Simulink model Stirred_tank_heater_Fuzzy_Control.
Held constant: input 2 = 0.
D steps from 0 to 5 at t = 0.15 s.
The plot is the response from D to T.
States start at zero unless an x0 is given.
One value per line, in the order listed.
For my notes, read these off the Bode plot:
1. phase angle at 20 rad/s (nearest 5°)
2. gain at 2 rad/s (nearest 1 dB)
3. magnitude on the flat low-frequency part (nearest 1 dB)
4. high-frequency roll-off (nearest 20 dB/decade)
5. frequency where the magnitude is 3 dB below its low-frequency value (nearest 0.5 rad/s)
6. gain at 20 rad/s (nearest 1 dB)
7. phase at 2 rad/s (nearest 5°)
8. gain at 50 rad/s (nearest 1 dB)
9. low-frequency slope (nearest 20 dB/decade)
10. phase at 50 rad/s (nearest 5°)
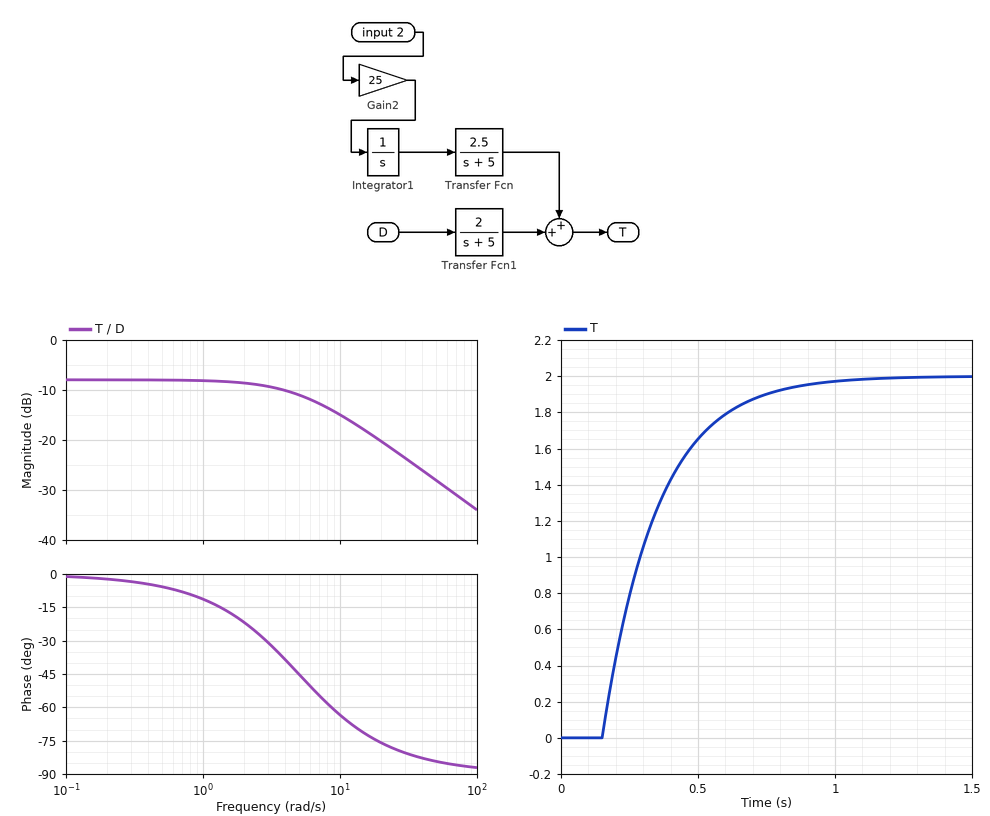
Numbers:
-75°
-9 dB
-8 dB
-20 dB/decade
5.0 rad/s
-20 dB
-20°
-28 dB
0 dB/decade
-85°
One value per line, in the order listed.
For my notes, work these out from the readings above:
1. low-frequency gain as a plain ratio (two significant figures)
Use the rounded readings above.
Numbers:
0.40
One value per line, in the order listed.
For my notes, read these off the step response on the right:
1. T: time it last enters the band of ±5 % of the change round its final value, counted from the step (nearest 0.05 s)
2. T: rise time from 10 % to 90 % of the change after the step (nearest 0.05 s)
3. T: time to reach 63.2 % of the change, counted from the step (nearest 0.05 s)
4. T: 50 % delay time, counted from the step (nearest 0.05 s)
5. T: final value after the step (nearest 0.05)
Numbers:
0.60 s
0.45 s
0.20 s
0.15 s
2.00
